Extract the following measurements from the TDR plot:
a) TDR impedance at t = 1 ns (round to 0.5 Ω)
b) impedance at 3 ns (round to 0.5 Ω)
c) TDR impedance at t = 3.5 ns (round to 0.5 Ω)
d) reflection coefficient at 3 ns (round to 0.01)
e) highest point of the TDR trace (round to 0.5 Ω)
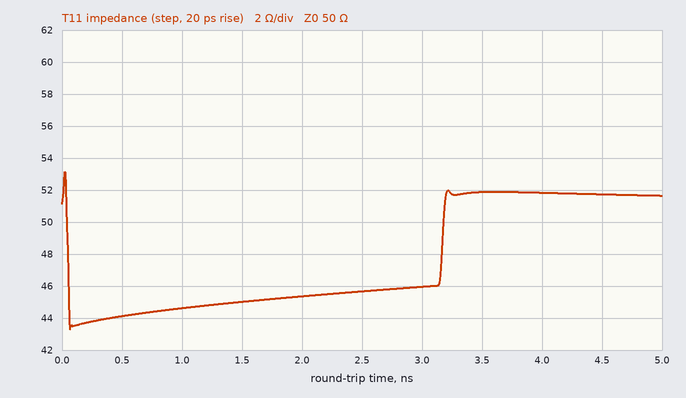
44.5 Ω
46.0 Ω
52.0 Ω
-0.04
53.0 Ω
